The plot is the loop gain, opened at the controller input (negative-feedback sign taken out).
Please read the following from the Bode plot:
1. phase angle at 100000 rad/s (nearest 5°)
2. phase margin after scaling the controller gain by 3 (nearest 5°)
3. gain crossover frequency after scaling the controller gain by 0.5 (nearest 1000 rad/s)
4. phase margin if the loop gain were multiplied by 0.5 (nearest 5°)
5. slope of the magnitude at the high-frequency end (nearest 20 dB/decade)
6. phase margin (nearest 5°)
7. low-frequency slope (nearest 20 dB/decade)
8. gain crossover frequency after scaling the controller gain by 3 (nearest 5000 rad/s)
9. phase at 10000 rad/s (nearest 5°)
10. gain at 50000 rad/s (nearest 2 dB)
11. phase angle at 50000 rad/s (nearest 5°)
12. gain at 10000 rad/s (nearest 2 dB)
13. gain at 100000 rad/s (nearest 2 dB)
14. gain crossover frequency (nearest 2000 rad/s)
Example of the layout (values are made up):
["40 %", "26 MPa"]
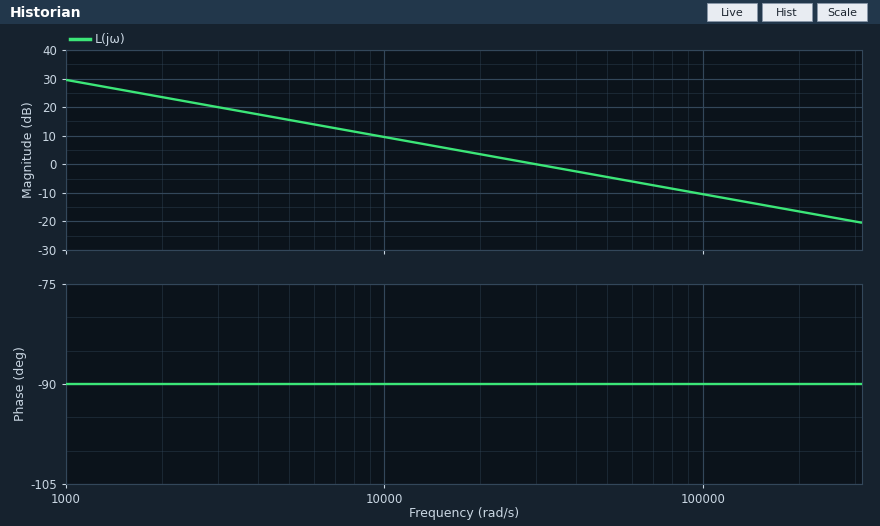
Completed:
["-90°", "90°", "15000 rad/s", "90°", "-20 dB/decade", "90°", "-20 dB/decade", "90000 rad/s", "-90°", "-4 dB", "-90°", "10 dB", "-10 dB", "30000 rad/s"]
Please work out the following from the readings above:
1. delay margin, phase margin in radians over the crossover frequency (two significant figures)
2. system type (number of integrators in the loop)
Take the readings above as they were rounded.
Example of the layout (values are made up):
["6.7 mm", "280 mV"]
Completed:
["0.000052 s", "1"]
